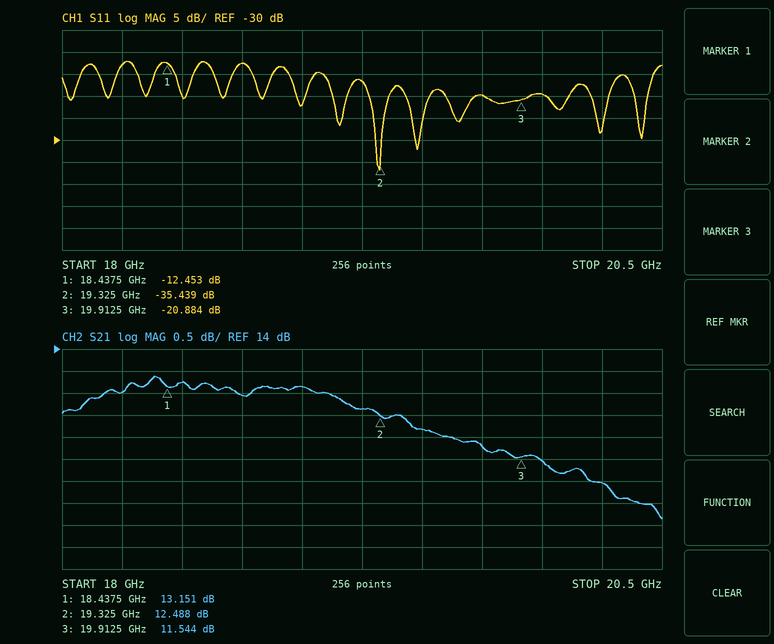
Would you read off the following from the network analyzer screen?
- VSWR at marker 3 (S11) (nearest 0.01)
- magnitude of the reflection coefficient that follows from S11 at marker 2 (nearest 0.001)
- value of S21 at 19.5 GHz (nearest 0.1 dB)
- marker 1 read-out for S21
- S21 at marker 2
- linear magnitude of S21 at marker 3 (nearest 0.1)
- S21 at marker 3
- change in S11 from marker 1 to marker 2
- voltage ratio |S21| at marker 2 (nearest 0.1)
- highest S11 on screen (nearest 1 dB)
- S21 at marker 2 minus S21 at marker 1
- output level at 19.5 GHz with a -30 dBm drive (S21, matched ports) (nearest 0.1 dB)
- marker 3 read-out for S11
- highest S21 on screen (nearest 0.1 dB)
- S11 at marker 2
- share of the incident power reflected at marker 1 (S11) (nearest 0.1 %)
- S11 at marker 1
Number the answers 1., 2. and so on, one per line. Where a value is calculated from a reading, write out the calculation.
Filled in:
1. (1 + 0.0903)/(1 − 0.0903) ≈ 1.20
2. 10^(-35.439/20) ≈ 0.017
3. 12.2 dB
4. 13.151 dB
5. 12.488 dB
6. 10^(11.544/20) ≈ 3.8
7. 11.544 dB
8. -35.439 − (-12.453) = -22.986 dB
9. 10^(12.488/20) ≈ 4.2
10. -12 dB
11. 12.488 − (13.151) = -0.663 dB
12. -30 dBm + (12.2 dB) = -17.8 dBm
13. -20.884 dB
14. 13.4 dB
15. -35.439 dB
16. 10^(-12.453/10) ≈ 5.7 %
17. -12.453 dB
